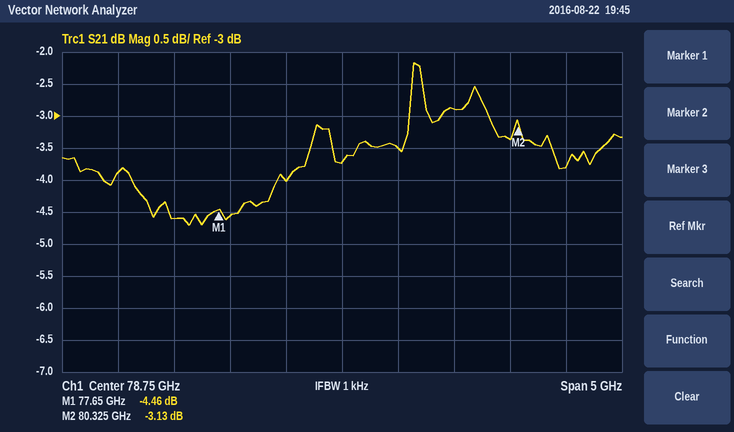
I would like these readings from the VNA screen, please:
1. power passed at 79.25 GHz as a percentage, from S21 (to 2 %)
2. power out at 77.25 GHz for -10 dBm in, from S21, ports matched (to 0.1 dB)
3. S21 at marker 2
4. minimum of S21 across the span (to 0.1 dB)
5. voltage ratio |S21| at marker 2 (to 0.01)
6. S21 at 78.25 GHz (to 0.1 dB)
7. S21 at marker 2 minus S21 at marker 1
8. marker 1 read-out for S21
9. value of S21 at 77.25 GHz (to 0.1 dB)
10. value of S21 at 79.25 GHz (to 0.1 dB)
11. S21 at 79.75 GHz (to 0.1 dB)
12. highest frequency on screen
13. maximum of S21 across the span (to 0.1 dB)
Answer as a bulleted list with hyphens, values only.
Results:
- 44 %
- -14.6 dBm
- -3.13 dB
- -4.7 dB
- 0.70
- -4.0 dB
- 1.33 dB
- -4.46 dB
- -4.6 dB
- -3.5 dB
- -2.9 dB
- 81.25 GHz
- -2.2 dB
